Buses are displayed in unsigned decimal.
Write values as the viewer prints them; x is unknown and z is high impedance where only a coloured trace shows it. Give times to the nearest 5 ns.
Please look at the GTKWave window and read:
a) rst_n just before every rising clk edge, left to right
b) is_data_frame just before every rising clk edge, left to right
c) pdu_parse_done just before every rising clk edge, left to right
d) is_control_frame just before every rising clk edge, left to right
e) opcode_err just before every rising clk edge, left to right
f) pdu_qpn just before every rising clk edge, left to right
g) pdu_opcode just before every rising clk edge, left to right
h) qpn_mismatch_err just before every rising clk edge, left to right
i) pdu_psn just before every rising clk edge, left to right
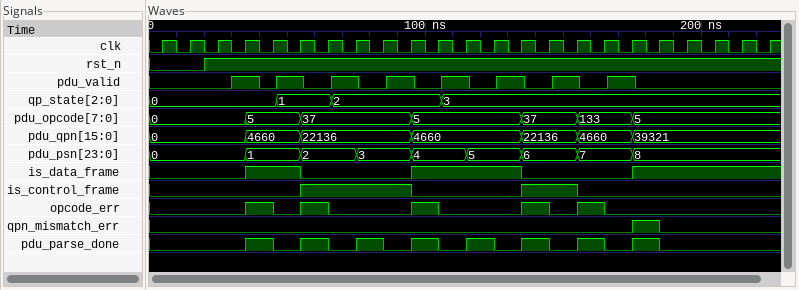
0 0 1 1 1 1 1 1 1 1 1 1 1 1 1 1 1 1 1 1 1 1 1
0 0 0 0 1 1 0 0 0 0 1 1 1 1 0 0 0 0 1 1 1 1 1
0 0 0 0 1 0 1 0 1 0 1 0 1 0 1 0 1 0 1 0 0 0 0
0 0 0 0 0 0 1 1 1 1 0 0 0 0 1 1 0 0 0 0 0 0 0
0 0 0 0 1 0 1 0 0 0 1 0 0 0 1 0 1 0 0 0 0 0 0
0, 0, 0, 0, 4660, 4660, 22136, 22136, 22136, 22136, 4660, 4660, 4660, 4660, 22136, 22136, 4660, 4660, 39321, 39321, 39321, 39321, 39321
0, 0, 0, 0, 5, 5, 37, 37, 37, 37, 5, 5, 5, 5, 37, 37, 133, 133, 5, 5, 5, 5, 5
0 0 0 0 0 0 0 0 0 0 0 0 0 0 0 0 0 0 1 0 0 0 0
0, 0, 0, 0, 1, 1, 2, 2, 3, 3, 4, 4, 5, 5, 6, 6, 7, 7, 8, 8, 8, 8, 8
